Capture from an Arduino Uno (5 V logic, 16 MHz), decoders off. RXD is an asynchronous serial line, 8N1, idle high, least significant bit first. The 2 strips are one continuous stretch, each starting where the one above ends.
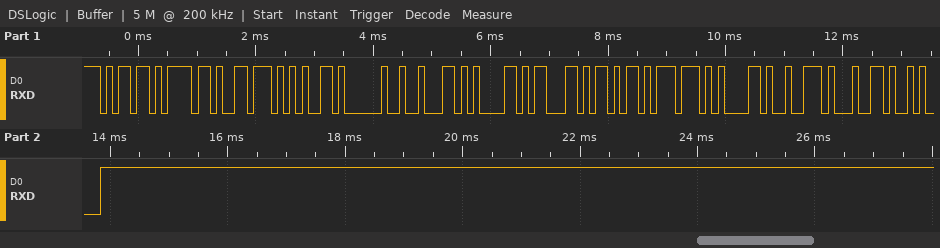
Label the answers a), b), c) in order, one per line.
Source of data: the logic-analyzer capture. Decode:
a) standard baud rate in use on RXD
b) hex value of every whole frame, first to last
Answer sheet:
a) 9600 baud
b) 0x6D 0x6F 0x76 0x65 0x20 0x62 0x61 0x63 0x6B 0x77 0x61 0x72 0x64 0x0A
